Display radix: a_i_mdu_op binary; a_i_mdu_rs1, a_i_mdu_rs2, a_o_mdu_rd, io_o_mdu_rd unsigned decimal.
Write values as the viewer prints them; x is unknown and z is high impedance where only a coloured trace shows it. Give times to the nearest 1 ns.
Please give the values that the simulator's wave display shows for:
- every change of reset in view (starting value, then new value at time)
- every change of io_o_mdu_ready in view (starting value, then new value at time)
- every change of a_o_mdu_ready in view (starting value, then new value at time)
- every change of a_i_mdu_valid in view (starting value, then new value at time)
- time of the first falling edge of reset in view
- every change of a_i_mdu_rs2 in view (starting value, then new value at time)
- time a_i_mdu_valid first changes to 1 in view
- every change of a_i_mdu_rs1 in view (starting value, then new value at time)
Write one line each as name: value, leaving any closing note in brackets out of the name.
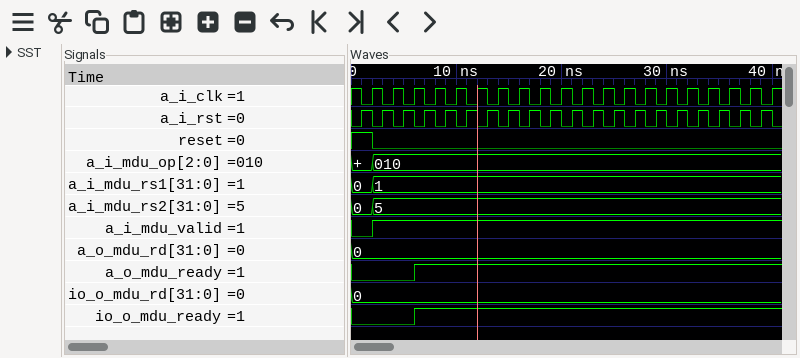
every change of reset in view: 1, 0 at 2 ns
every change of io_o_mdu_ready in view: 0, 1 at 6 ns
every change of a_o_mdu_ready in view: 0, 1 at 6 ns
every change of a_i_mdu_valid in view: 0, 1 at 2 ns
time of the first falling edge of reset in view: 2 ns
every change of a_i_mdu_rs2 in view: 0, 5 at 2 ns
time a_i_mdu_valid first changes to 1 in view: 2 ns
every change of a_i_mdu_rs1 in view: 0, 1 at 2 ns
